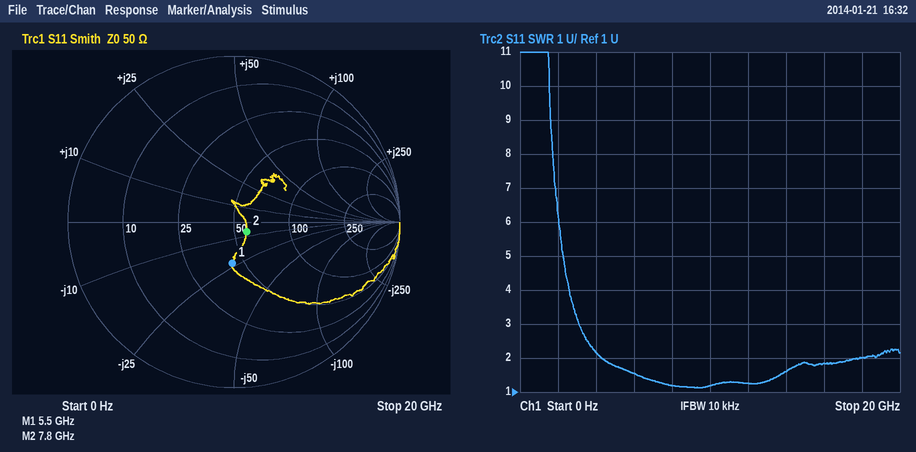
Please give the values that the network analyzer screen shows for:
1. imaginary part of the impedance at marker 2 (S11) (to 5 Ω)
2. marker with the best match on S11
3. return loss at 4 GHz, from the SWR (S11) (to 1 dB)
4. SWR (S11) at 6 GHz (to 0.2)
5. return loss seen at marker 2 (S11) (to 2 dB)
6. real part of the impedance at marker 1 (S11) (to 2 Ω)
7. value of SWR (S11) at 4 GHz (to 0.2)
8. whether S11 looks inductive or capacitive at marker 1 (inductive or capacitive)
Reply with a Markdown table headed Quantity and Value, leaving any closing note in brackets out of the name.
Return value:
| Quantity | Value |
|---|---|
| imaginary part of the impedance at marker 2 (S11) | -5 Ω |
| marker with the best match on S11 | marker 2 |
| return loss at 4 GHz, from the SWR (S11) | 9 dB |
| SWR (S11) at 6 GHz | 1.6 |
| return loss seen at marker 2 (S11) | 20 dB |
| real part of the impedance at marker 1 (S11) | 44 Ω |
| value of SWR (S11) at 4 GHz | 2.2 |
| whether S11 looks inductive or capacitive at marker 1 | capacitive |
